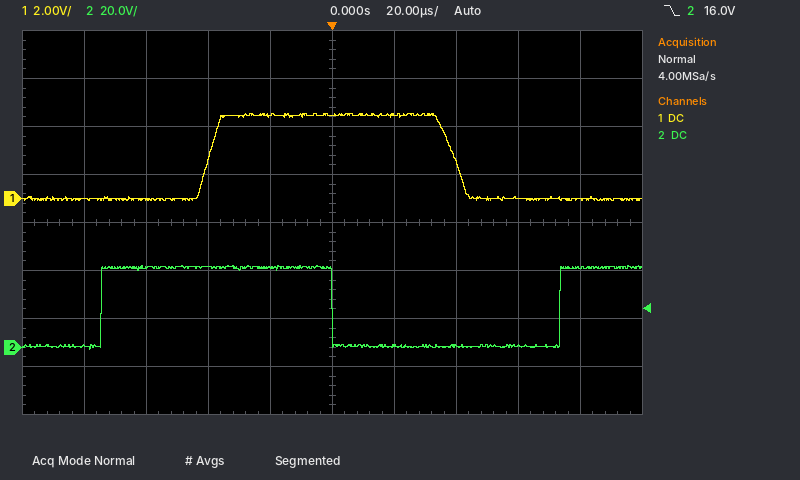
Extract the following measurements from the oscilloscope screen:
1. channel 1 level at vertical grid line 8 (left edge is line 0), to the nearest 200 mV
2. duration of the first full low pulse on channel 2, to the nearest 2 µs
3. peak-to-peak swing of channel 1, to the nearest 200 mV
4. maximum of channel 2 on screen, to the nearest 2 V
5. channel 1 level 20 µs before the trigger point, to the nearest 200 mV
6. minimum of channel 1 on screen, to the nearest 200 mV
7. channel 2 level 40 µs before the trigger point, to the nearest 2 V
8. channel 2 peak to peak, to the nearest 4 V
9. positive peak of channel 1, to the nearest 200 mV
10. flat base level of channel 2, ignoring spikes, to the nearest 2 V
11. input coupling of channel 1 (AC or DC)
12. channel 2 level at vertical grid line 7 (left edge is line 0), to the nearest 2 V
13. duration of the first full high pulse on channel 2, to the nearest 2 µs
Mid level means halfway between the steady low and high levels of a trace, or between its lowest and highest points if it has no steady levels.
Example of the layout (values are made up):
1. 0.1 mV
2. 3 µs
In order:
1. 0.0 V
2. 74 µs
3. 3.6 V
4. 34 V
5. 3.4 V
6. 0.0 V
7. 34 V
8. 36 V
9. 3.6 V
10. 0 V
11. DC
12. 0 V
13. 74 µs
